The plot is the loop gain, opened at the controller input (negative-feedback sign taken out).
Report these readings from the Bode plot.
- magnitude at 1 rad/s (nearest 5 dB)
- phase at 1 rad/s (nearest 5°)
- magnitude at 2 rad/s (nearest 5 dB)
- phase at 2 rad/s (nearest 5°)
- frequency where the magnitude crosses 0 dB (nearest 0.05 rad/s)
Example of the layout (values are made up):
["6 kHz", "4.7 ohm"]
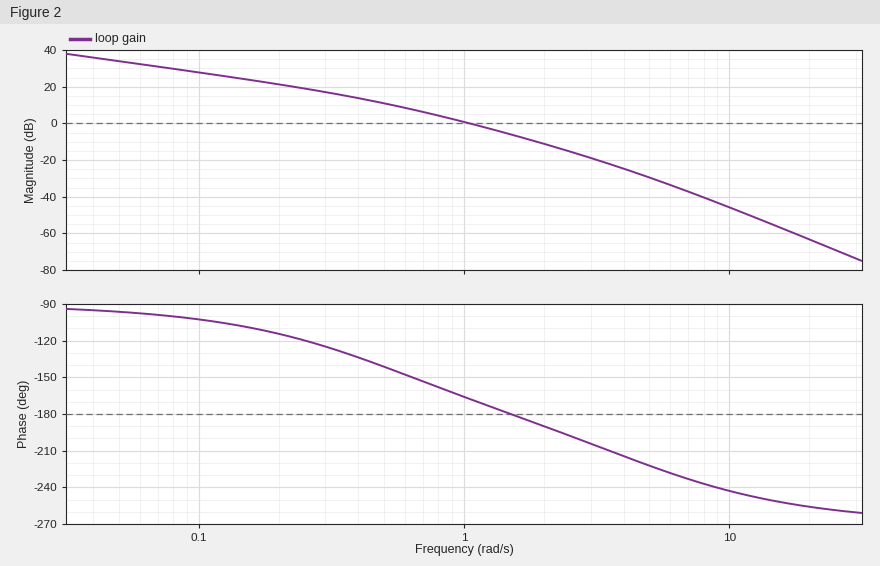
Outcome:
["0 dB", "-165°", "-10 dB", "-190°", "1.05 rad/s"]
